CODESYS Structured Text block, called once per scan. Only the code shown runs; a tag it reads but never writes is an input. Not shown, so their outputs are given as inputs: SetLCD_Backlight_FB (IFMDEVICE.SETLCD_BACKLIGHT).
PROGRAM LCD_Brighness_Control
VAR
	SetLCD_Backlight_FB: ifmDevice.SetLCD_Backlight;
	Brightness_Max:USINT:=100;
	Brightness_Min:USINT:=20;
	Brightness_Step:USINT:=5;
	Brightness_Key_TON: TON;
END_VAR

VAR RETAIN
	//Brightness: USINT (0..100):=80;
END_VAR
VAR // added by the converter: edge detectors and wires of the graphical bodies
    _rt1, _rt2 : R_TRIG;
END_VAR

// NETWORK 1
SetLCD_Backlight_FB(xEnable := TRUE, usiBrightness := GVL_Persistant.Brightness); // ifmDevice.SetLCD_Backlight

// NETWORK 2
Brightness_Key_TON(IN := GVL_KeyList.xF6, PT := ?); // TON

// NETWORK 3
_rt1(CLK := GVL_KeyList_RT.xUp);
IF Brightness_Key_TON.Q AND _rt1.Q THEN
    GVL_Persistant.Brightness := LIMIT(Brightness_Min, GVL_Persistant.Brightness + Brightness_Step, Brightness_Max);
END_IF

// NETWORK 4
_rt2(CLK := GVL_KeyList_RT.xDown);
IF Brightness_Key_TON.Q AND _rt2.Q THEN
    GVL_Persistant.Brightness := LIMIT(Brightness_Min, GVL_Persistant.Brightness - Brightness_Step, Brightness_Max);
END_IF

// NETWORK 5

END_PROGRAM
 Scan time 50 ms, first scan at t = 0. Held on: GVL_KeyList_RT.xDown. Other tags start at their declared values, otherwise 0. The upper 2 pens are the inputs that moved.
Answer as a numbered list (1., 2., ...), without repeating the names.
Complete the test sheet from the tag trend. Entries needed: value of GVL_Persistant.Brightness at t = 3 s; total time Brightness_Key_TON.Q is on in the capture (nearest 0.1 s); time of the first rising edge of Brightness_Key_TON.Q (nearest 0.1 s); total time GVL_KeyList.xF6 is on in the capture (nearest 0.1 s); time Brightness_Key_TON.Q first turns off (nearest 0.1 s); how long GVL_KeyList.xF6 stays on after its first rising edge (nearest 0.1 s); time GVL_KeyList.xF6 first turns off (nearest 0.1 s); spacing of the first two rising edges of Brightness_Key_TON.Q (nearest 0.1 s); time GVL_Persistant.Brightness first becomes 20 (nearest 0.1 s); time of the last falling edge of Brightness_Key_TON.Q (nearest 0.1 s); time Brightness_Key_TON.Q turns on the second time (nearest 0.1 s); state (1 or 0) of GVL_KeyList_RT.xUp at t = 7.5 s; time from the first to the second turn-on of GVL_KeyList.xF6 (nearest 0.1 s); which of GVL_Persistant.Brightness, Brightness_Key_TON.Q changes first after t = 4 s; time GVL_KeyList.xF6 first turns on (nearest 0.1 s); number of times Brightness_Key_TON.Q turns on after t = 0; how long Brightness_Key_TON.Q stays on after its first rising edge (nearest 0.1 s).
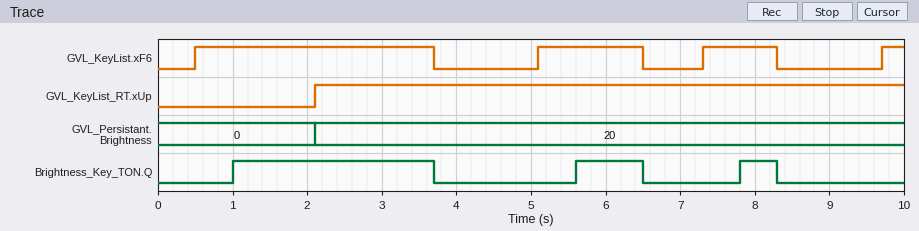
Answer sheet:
1. 20
2. 4.1 s
3. 1.0 s
4. 5.9 s
5. 3.7 s
6. 3.2 s
7. 3.7 s
8. 4.6 s
9. 2.1 s
10. 8.3 s
11. 5.6 s
12. 1
13. 4.6 s
14. Brightness_Key_TON.Q
15. 0.5 s
16. 3
17. 2.7 s
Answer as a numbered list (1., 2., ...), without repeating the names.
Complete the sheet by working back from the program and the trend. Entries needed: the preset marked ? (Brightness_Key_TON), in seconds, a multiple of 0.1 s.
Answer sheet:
1. 0.5 s
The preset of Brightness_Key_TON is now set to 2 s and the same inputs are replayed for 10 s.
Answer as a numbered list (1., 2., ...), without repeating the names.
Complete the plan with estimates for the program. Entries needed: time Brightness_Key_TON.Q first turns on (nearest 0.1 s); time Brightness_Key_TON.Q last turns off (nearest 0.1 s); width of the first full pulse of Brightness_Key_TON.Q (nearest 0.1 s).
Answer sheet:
1. 2.5 s
2. 3.7 s
3. 1.2 s
